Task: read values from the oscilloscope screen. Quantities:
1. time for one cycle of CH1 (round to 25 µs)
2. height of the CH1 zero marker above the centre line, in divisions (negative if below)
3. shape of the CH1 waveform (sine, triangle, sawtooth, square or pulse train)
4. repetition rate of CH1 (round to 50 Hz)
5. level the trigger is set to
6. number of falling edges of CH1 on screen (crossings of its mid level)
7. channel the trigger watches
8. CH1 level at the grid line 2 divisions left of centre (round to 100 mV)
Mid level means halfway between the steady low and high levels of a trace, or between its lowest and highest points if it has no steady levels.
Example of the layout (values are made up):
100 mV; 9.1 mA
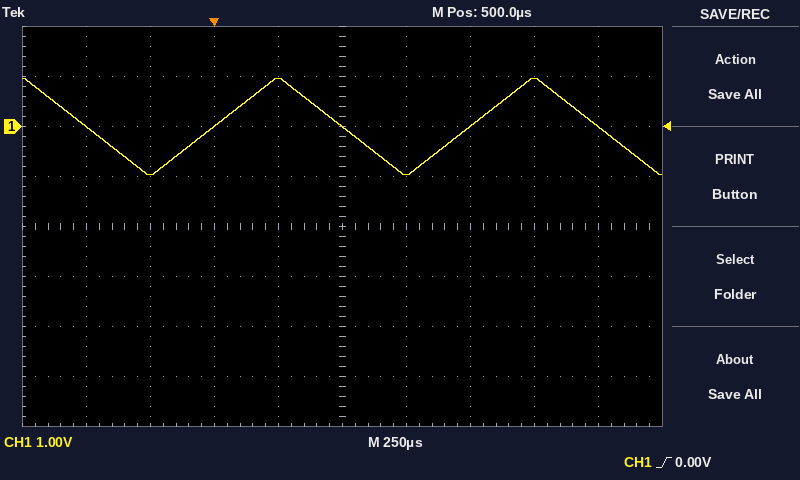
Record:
1.000 ms; +2.0 div; triangle; 1.00 kHz; 0.00 V; 3; CH1; 0.0 V
